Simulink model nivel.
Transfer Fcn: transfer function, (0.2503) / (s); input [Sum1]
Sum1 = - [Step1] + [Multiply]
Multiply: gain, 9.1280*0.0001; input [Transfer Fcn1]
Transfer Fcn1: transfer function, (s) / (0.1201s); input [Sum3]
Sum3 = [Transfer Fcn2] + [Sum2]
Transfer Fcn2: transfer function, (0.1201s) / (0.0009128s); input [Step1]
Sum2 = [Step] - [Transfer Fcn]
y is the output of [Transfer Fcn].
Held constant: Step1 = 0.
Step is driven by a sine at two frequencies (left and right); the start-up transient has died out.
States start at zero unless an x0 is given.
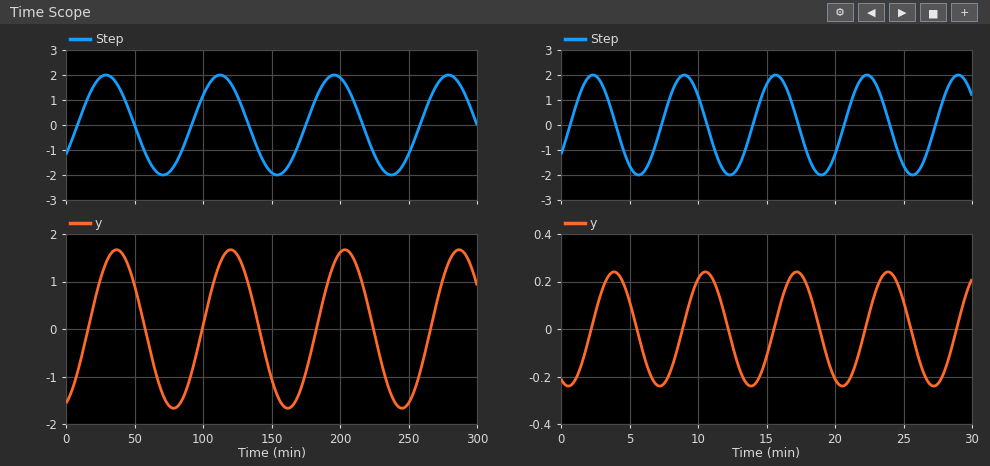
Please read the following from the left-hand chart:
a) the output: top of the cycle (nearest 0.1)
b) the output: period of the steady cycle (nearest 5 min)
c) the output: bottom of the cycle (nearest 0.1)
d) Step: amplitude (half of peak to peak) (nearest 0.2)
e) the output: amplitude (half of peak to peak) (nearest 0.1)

1.7
85 min
-1.7
2.0
1.7
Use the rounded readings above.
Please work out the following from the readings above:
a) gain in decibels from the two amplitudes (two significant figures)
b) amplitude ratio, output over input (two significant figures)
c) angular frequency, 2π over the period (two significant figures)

-1.4 dB
0.85
0.074 rad/min
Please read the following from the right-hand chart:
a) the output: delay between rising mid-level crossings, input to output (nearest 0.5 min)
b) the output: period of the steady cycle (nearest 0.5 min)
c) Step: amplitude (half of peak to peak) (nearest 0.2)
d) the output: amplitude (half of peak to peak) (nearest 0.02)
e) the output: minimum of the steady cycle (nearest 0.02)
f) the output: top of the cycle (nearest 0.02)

1.5 min
6.5 min
2.0
0.24
-0.24
0.24
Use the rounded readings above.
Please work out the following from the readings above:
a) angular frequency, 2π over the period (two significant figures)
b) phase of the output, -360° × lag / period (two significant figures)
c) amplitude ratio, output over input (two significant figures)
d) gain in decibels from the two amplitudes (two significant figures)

0.97 rad/min
-83°
0.12
-18 dB
